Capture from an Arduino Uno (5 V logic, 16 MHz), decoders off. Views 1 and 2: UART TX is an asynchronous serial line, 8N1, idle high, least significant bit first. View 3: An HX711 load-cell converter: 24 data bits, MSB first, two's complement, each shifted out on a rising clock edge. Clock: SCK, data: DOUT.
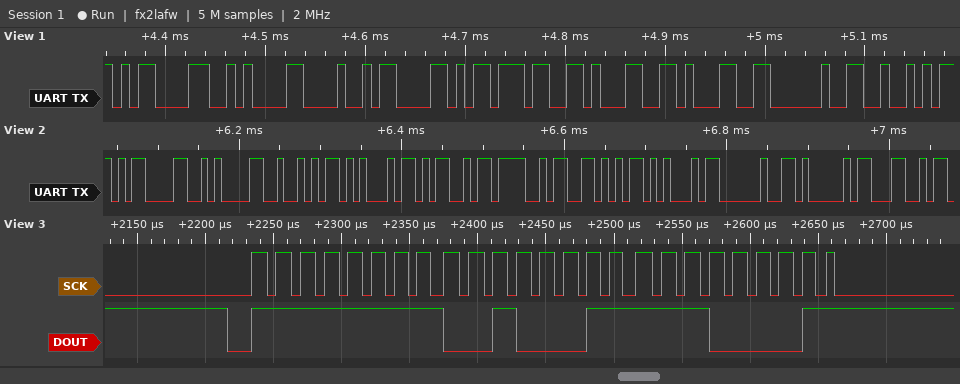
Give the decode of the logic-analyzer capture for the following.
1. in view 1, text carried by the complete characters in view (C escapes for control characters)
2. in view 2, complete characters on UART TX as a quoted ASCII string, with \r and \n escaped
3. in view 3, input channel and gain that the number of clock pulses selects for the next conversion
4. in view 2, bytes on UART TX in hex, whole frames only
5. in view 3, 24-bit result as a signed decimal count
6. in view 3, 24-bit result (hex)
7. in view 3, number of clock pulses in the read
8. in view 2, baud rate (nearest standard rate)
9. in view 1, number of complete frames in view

"\r\nHX711 R"
"\r\nREMOVE AL"
channel A, gain 128
0x0D 0x0A 0x52 0x45 0x4D 0x4F 0x56 0x45 0x20 0x41 0x4C
-56351
0xFF23E1
25
115200 baud
9
